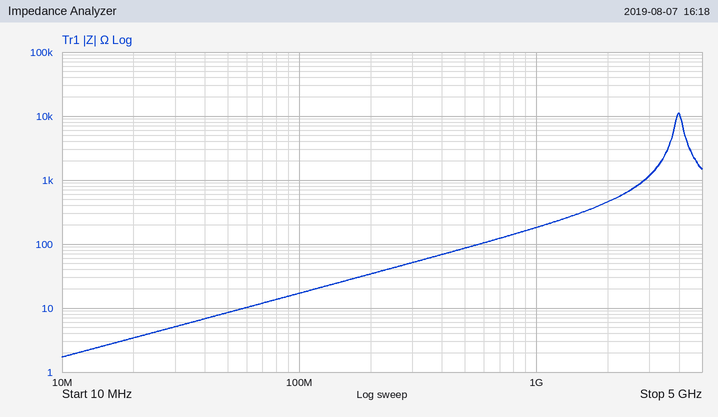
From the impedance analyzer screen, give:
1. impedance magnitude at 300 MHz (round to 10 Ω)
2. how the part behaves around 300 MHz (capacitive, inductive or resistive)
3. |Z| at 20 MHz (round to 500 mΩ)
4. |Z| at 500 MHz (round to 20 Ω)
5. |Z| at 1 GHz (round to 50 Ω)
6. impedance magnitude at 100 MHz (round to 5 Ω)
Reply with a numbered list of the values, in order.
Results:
1. 50 Ω
2. inductive
3. 3.5 Ω
4. 80 Ω
5. 200 Ω
6. 15 Ω
